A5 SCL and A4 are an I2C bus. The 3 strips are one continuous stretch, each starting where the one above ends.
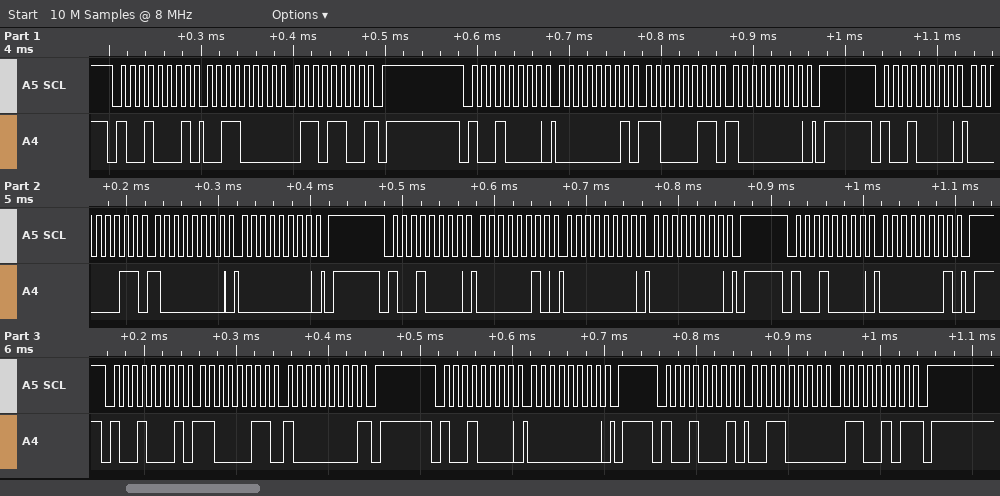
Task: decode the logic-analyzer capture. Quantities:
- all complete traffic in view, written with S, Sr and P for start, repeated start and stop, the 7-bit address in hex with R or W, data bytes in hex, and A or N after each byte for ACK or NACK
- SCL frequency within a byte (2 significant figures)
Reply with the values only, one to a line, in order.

S 48R A 30 A 6C N P S 48W A 01 A C3 A 80 A P S 48W A 03 A 80 A 00 A P S 48W A 02 A 00 A 00 A P S 48W A 01 A P S 48R A C3 A 80 N P S 48W A 00 A P S 48R A 30 A 65 N P
100 kHz
